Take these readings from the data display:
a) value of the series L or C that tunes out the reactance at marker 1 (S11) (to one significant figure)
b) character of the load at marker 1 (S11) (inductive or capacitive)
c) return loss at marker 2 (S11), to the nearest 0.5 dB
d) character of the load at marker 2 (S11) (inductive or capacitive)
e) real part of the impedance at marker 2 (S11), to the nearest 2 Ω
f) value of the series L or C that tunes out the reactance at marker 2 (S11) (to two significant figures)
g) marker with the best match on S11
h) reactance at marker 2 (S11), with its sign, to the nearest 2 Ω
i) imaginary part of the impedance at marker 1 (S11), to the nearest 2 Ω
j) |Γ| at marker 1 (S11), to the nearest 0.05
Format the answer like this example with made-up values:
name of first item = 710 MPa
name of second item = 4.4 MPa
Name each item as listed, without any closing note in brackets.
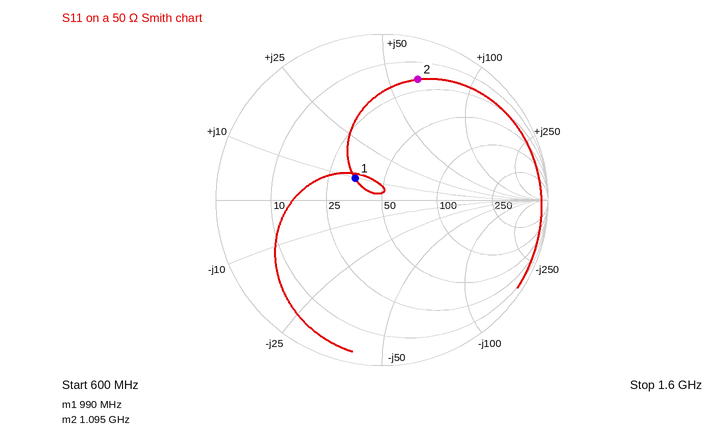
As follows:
value of the series L or C that tunes out the reactance at marker 1 (S11) = 20 pF
character of the load at marker 1 (S11) = inductive
return loss at marker 2 (S11), to the nearest 0.5 dB = 2.5 dB
character of the load at marker 2 (S11) = inductive
real part of the impedance at marker 2 (S11), to the nearest 2 Ω = 18 Ω
value of the series L or C that tunes out the reactance at marker 2 (S11) = 2.3 pF
marker with the best match on S11 = marker 1
reactance at marker 2 (S11), with its sign, to the nearest 2 Ω = +64 Ω
imaginary part of the impedance at marker 1 (S11), to the nearest 2 Ω = +10 Ω
|Γ| at marker 1 (S11), to the nearest 0.05 = 0.20
